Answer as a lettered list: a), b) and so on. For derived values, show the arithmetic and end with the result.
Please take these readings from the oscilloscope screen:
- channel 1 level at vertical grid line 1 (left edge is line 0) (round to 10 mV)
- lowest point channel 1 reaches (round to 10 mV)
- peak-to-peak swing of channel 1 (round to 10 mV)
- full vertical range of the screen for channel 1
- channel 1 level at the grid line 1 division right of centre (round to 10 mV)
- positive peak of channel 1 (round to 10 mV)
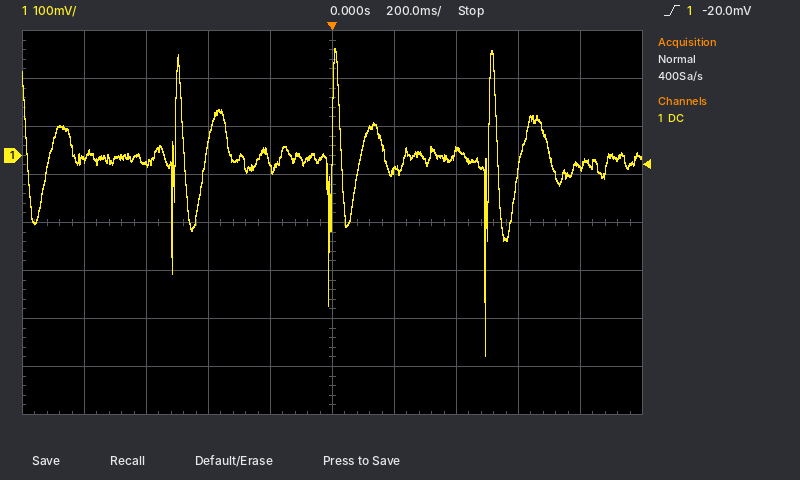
a) -10 mV
b) -420 mV
c) 220 mV − (-420 mV) = 640 mV
d) 800 mV
e) -30 mV
f) 220 mV
